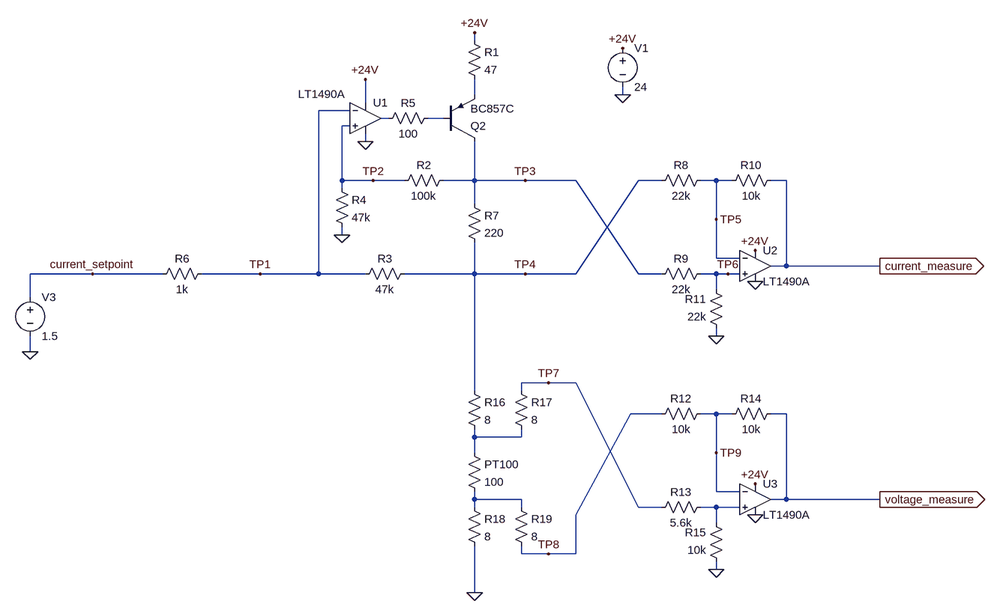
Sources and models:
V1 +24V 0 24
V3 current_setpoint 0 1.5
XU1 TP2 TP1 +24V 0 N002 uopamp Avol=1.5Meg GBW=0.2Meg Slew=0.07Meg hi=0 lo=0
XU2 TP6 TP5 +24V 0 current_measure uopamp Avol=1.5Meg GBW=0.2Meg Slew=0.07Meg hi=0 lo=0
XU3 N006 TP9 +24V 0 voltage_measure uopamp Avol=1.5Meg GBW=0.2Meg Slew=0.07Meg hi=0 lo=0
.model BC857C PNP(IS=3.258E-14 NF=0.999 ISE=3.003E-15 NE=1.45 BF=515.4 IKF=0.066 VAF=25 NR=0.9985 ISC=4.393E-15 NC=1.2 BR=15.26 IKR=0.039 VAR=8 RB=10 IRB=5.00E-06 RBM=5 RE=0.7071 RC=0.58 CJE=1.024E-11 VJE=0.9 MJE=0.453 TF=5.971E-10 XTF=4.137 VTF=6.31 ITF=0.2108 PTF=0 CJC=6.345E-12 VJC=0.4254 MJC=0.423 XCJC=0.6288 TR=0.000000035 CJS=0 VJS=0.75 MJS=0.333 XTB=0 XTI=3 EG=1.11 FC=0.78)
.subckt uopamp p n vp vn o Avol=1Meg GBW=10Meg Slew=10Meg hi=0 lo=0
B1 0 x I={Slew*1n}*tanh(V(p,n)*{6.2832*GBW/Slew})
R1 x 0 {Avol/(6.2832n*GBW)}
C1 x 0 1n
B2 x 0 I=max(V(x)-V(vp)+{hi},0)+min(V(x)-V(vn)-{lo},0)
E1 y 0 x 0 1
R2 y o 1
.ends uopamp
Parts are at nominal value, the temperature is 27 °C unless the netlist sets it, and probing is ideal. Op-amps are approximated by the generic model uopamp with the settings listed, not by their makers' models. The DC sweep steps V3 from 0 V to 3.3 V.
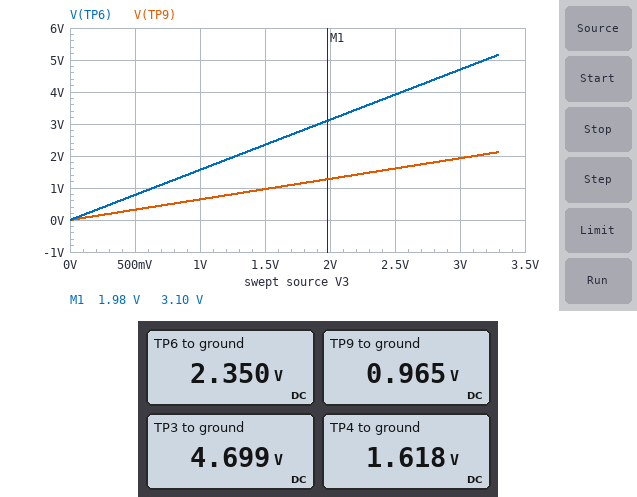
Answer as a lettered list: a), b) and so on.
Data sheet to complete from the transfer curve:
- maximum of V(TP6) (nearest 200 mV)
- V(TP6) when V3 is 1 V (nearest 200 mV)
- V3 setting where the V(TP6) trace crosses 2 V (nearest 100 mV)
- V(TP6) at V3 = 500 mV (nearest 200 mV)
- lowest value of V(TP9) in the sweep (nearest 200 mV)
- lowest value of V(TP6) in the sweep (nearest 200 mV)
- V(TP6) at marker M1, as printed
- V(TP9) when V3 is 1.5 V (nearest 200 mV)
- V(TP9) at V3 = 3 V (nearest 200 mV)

a) 5.2 V
b) 1.6 V
c) 1.3 V
d) 800 mV
e) 0 V
f) 0 V
g) 3.10 V
h) 1.0 V
i) 2.0 V
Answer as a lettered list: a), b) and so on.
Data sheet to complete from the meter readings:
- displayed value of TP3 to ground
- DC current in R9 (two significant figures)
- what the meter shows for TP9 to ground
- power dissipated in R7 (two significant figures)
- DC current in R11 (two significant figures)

a) 4.699 V
b) 110 µA
c) 0.965 V
d) 43 mW
e) 110 µA
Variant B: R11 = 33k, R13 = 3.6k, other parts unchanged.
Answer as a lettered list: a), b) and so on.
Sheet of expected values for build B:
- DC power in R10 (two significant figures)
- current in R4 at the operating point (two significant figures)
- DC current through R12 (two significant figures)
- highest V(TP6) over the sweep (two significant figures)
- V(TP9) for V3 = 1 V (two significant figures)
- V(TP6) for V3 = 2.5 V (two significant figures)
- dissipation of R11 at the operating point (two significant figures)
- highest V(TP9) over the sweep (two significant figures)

a) 30 µW
b) 32 µA
c) 99 µA
d) 6.2 V
e) 740 mV
f) 4.7 V
g) 240 µW
h) 2.4 V
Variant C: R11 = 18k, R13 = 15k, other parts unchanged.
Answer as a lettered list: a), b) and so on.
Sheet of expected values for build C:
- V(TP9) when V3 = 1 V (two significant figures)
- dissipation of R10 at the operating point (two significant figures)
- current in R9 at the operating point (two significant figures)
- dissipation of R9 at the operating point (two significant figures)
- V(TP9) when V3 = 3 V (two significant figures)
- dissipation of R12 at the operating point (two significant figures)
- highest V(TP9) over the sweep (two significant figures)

a) 400 mV
b) 5.1 µW
c) 120 µA
d) 300 µW
e) 1.2 V
f) 24 µW
g) 1.3 V
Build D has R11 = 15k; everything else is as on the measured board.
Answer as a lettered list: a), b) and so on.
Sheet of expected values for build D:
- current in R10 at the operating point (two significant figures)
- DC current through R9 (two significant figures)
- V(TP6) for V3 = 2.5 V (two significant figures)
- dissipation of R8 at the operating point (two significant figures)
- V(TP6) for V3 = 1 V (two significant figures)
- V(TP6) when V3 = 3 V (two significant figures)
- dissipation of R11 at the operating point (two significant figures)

a) 13 µA
b) 130 µA
c) 3.2 V
d) 3.8 µW
e) 1.3 V
f) 3.8 V
g) 240 µW
